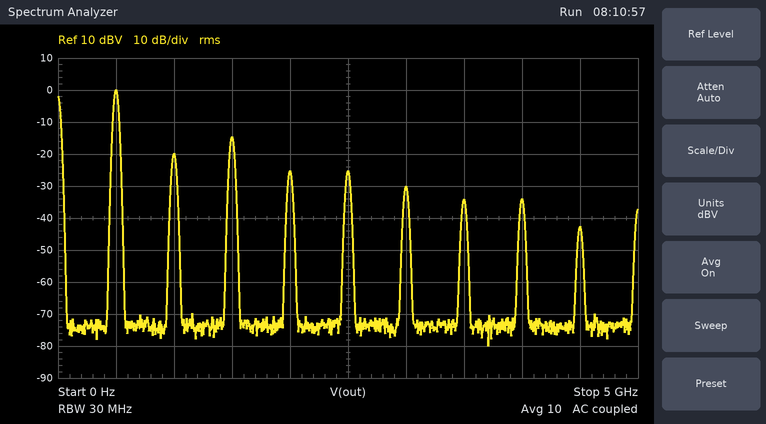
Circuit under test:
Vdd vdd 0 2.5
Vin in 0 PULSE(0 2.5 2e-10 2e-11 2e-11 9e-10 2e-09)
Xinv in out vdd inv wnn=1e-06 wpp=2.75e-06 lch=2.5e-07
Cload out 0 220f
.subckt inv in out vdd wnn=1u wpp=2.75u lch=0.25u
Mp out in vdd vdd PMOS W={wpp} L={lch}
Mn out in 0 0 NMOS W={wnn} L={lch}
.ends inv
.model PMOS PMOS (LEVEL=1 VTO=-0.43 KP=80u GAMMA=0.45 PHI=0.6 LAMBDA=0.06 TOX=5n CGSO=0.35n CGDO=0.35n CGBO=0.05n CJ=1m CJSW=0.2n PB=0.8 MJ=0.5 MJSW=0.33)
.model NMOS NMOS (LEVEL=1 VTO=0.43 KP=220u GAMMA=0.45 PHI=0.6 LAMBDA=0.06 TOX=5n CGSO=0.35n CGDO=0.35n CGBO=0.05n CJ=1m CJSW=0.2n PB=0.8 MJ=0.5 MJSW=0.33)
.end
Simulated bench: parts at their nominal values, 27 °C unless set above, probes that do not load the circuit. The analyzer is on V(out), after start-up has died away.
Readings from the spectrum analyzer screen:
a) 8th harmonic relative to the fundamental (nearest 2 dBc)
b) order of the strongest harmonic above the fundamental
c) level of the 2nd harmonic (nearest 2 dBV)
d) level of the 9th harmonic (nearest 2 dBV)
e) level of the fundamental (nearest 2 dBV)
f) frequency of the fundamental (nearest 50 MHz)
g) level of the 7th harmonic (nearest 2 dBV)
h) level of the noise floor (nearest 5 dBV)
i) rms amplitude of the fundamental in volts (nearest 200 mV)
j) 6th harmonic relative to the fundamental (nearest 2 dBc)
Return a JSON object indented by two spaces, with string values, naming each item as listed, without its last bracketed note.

{
  "8th harmonic relative to the fundamental": "-34 dBc",
  "order of the strongest harmonic above the fundamental": "3",
  "level of the 2nd harmonic": "-20 dBV",
  "level of the 9th harmonic": "-42 dBV",
  "level of the fundamental": "0 dBV",
  "frequency of the fundamental": "500 MHz",
  "level of the 7th harmonic": "-34 dBV",
  "level of the noise floor": "-75 dBV",
  "rms amplitude of the fundamental in volts": "1.0 V",
  "6th harmonic relative to the fundamental": "-30 dBc"
}
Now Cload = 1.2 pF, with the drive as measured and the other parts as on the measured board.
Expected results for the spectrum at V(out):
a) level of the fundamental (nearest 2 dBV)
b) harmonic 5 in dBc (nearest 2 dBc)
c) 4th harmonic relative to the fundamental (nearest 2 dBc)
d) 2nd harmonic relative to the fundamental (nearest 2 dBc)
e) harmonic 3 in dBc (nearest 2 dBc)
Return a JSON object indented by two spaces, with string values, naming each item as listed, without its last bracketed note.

{
  "level of the fundamental": "-8 dBV",
  "harmonic 5 in dBc": "-30 dBc",
  "4th harmonic relative to the fundamental": "-30 dBc",
  "2nd harmonic relative to the fundamental": "-24 dBc",
  "harmonic 3 in dBc": "-20 dBc"
}
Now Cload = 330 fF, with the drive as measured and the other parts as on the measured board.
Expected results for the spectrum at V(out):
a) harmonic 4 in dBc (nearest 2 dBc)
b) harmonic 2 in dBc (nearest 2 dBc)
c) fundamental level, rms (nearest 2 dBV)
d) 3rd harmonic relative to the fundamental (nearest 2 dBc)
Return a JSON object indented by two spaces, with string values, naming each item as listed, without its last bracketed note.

{
  "harmonic 4 in dBc": "-28 dBc",
  "harmonic 2 in dBc": "-22 dBc",
  "fundamental level, rms": "0 dBV",
  "3rd harmonic relative to the fundamental": "-18 dBc"
}
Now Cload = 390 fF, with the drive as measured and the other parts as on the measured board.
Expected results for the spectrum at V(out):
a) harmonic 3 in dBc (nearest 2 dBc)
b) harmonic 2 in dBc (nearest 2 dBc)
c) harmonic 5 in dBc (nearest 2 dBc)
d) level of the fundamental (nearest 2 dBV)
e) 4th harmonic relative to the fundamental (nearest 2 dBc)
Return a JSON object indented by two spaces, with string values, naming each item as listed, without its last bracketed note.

{
  "harmonic 3 in dBc": "-18 dBc",
  "harmonic 2 in dBc": "-22 dBc",
  "harmonic 5 in dBc": "-30 dBc",
  "level of the fundamental": "-2 dBV",
  "4th harmonic relative to the fundamental": "-30 dBc"
}
